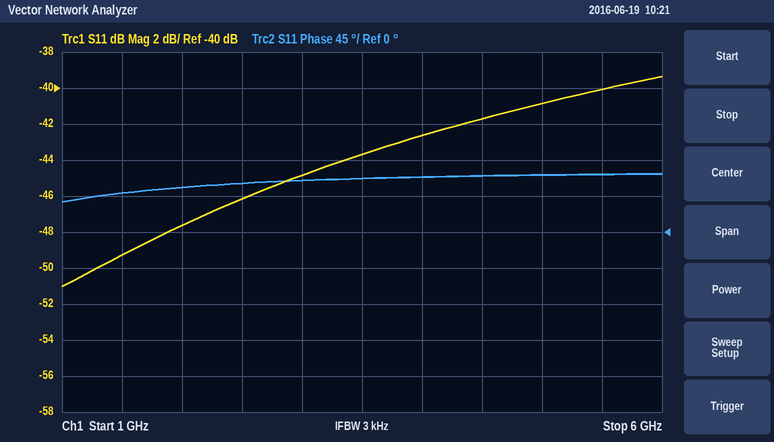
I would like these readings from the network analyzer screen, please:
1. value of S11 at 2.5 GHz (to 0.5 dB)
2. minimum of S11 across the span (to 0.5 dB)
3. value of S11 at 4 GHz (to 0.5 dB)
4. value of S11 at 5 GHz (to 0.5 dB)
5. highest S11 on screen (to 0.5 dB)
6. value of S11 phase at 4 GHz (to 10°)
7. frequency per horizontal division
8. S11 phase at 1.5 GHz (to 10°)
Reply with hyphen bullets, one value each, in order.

- -46.0 dB
- -51.0 dB
- -42.5 dB
- -41.0 dB
- -39.5 dB
- 70°
- 500 MHz
- 50°
